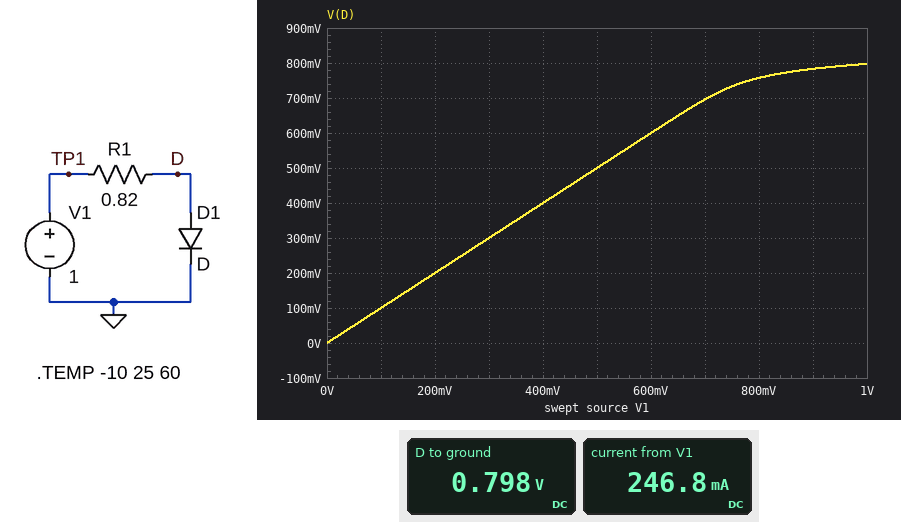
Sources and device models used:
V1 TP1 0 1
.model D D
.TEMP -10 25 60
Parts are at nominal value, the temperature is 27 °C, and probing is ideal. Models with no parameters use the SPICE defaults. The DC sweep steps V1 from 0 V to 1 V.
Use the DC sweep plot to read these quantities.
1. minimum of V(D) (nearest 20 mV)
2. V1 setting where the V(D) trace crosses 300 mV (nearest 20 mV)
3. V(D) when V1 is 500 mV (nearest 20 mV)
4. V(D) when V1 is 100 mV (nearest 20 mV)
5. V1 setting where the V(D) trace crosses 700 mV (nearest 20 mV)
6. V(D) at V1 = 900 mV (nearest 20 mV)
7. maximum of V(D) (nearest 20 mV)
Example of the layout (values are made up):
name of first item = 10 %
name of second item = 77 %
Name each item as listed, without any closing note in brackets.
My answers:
minimum of V(D) = 0 V
V1 setting where the V(D) trace crosses 300 mV = 300 mV
V(D) when V1 is 500 mV = 500 mV
V(D) when V1 is 100 mV = 100 mV
V1 setting where the V(D) trace crosses 700 mV = 700 mV
V(D) at V1 = 900 mV = 780 mV
maximum of V(D) = 800 mV
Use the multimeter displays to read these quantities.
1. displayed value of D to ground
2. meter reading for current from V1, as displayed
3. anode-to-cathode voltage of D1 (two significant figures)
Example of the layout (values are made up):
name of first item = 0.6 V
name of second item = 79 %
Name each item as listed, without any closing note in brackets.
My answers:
displayed value of D to ground = 0.798 V
meter reading for current from V1, as displayed = 246.8 mA
anode-to-cathode voltage of D1 = 800 mV
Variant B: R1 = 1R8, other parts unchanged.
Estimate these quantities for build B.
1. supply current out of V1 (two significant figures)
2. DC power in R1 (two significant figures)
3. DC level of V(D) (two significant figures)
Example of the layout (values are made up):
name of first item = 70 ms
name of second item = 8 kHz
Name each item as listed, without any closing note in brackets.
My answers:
supply current out of V1 = 120 mA
DC power in R1 = 27 mW
DC level of V(D) = 780 mV
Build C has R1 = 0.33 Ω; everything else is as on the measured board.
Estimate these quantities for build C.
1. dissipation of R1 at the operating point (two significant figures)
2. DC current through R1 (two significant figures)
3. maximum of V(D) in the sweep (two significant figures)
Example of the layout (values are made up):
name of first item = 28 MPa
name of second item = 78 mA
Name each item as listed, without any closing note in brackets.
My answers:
dissipation of R1 at the operating point = 100 mW
DC current through R1 = 550 mA
maximum of V(D) in the sweep = 820 mV
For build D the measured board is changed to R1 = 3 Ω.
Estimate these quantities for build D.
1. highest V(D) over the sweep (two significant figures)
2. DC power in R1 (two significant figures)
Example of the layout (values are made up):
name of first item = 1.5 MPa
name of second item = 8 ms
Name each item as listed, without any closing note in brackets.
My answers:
highest V(D) over the sweep = 770 mV
DC power in R1 = 18 mW
